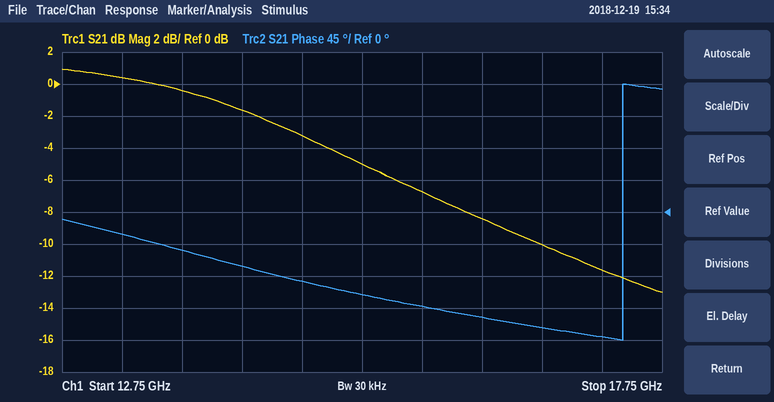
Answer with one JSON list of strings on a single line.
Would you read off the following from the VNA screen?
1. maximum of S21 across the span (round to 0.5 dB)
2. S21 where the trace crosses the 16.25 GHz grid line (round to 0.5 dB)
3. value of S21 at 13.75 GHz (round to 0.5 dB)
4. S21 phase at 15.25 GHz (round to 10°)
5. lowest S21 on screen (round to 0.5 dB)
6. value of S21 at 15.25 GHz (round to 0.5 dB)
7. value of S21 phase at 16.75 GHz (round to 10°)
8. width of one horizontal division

["1.0 dB", "-8.5 dB", "-0.5 dB", "-120°", "-13.0 dB", "-5.0 dB", "-160°", "500 MHz"]
